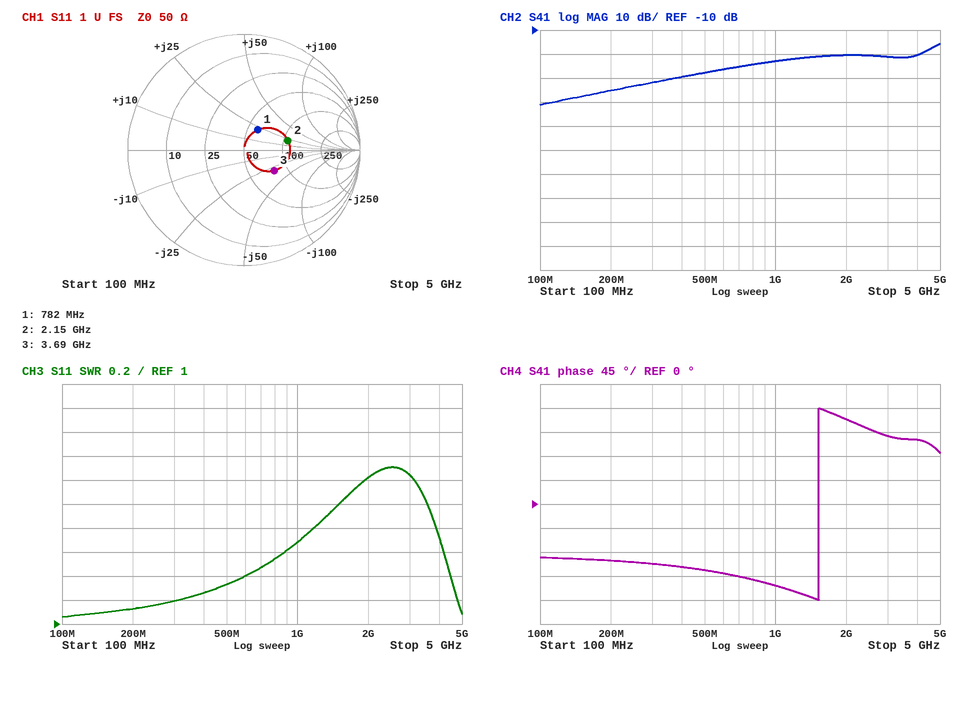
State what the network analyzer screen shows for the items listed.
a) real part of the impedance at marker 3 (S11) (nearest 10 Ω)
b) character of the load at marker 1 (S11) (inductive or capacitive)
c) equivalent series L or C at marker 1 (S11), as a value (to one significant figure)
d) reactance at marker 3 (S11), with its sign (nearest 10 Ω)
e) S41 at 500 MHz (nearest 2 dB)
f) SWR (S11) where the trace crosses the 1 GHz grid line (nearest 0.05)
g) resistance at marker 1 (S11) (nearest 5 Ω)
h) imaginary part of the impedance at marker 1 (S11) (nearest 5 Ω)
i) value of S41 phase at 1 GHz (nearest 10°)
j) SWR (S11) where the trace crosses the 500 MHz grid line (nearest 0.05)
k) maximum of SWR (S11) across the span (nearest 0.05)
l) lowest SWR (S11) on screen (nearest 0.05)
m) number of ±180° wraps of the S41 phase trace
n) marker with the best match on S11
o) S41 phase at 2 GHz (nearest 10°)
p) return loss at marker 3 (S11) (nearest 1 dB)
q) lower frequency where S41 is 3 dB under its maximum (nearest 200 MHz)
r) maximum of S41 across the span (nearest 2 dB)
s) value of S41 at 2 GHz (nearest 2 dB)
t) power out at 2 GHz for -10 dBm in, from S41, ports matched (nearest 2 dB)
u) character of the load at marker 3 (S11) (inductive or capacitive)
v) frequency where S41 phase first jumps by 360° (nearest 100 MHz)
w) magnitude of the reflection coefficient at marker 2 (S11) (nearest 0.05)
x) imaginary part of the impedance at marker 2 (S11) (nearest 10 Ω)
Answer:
80 Ω
inductive
4 nH
-30 Ω
-28 dB
1.70
60 Ω
+20 Ω
-150°
1.35
2.30
1.05
1
marker 1
160°
10 dB
4.4 GHz
-16 dB
-20 dB
-30 dBm
capacitive
1.5 GHz
0.40
+20 Ω
